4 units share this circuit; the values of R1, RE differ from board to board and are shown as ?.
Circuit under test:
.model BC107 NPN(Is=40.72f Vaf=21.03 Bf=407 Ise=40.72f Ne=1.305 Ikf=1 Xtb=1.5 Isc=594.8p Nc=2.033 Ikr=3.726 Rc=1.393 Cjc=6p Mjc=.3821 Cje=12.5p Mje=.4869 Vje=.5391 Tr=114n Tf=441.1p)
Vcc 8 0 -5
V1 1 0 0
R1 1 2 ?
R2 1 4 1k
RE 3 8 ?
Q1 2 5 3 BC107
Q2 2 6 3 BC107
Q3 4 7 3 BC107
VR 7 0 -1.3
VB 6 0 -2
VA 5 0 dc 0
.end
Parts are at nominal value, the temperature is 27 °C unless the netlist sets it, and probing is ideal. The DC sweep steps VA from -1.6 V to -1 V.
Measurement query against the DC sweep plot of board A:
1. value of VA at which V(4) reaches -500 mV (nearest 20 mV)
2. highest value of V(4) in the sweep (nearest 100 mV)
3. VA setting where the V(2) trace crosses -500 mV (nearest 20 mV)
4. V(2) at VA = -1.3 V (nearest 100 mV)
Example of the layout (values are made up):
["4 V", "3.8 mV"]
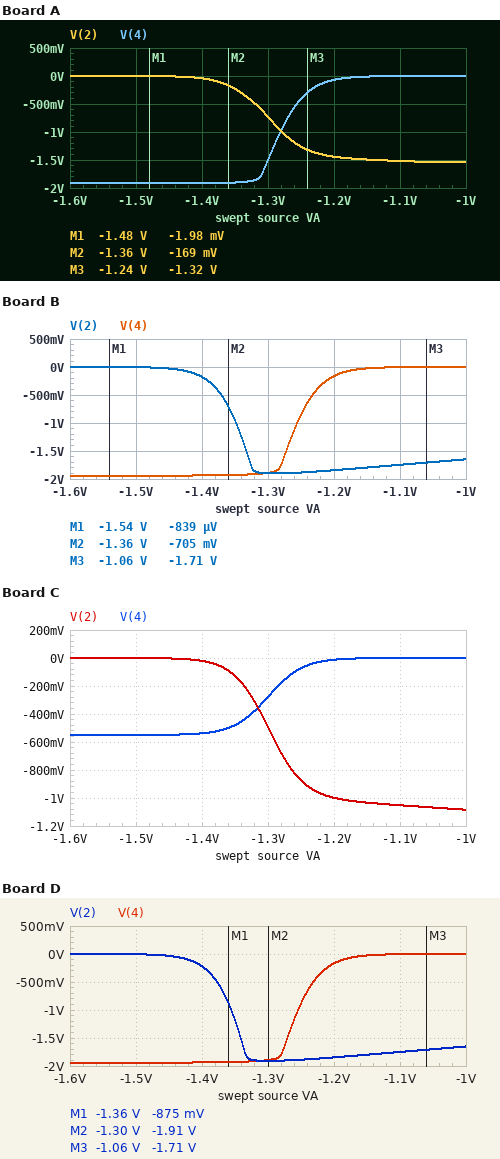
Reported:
["-1.26 V", "0 V", "-1.32 V", "-700 mV"]
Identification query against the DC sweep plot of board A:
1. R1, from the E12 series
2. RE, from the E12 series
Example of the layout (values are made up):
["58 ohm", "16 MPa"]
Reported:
["470 Ω", "1 kΩ"]
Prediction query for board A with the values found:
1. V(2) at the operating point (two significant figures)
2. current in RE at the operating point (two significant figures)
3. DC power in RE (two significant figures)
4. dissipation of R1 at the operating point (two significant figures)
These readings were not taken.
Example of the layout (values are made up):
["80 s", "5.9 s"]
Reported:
["-640 mV", "4.3 mA", "19 mW", "880 µW"]
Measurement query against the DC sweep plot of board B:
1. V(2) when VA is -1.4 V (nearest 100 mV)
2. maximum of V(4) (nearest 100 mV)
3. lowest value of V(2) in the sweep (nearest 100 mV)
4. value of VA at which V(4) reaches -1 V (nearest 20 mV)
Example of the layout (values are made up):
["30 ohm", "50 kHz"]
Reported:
["-200 mV", "0 V", "-1.9 V", "-1.26 V"]
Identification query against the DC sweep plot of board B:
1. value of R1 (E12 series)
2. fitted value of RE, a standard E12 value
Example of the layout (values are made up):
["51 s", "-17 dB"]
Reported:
["1.2 kΩ", "680 Ω"]
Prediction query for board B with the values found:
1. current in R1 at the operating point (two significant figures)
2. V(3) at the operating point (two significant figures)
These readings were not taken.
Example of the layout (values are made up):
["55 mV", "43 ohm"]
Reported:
["550 µA", "-680 mV"]
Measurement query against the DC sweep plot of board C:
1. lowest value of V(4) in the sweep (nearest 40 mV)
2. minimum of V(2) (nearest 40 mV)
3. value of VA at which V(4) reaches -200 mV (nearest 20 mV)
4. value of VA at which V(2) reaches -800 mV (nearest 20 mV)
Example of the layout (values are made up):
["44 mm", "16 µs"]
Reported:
["-560 mV", "-1.08 V", "-1.28 V", "-1.26 V"]
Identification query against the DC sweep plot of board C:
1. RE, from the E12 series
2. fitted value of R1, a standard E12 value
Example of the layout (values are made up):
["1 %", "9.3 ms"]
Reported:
["5.6 kΩ", "1.8 kΩ"]
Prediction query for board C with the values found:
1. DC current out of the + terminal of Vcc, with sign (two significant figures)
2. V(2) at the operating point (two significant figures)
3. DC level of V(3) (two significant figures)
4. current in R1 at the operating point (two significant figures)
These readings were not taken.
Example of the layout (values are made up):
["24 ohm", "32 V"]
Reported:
["-780 µA", "-590 mV", "-620 mV", "330 µA"]
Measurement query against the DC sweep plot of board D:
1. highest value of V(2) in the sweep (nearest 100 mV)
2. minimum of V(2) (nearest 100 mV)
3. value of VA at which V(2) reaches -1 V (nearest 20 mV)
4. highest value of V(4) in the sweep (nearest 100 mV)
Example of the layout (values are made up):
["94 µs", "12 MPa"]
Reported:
["0 V", "-1.9 V", "-1.36 V", "0 V"]
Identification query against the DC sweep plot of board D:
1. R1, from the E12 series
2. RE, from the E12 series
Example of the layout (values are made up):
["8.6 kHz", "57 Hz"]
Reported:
["1.5 kΩ", "680 Ω"]
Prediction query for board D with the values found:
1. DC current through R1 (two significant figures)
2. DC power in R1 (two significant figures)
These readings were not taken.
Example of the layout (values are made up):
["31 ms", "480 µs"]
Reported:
["440 µA", "290 µW"]
